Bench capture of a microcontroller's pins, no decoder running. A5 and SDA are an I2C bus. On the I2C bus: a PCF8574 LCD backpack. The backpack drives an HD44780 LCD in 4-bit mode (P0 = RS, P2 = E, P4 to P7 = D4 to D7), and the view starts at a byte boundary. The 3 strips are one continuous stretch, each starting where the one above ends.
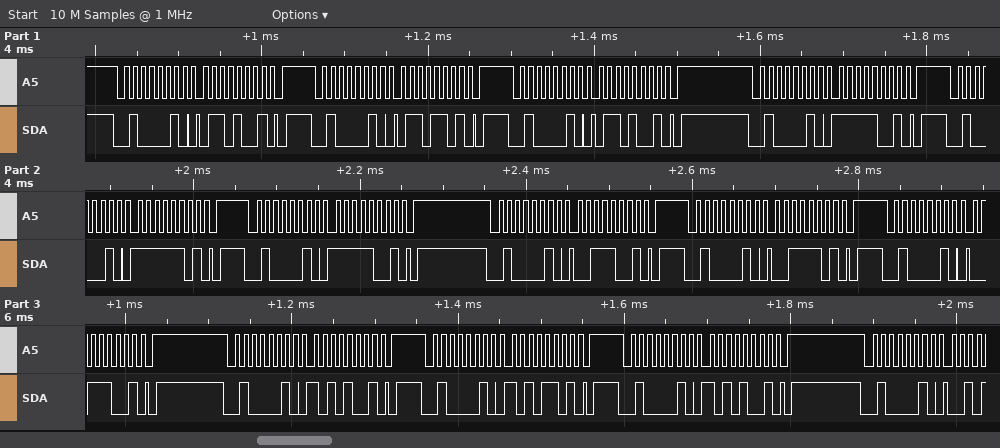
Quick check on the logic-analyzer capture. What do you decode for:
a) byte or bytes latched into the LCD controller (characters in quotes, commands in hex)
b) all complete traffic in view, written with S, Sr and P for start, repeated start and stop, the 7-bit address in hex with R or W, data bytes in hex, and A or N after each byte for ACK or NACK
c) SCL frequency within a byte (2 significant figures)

'o' ':'
S 21W A 69 A P S 21W A 6D A P S 21W A 69 A P S 21W A F9 A P S 21W A FD A P S 21W A F9 A P S 21W A 39 A P S 21W A 3D A P S 21W A 39 A P S 21W A A9 A P S 21W A AD A P S 21W A A9 A P S 21W A
100 kHz
